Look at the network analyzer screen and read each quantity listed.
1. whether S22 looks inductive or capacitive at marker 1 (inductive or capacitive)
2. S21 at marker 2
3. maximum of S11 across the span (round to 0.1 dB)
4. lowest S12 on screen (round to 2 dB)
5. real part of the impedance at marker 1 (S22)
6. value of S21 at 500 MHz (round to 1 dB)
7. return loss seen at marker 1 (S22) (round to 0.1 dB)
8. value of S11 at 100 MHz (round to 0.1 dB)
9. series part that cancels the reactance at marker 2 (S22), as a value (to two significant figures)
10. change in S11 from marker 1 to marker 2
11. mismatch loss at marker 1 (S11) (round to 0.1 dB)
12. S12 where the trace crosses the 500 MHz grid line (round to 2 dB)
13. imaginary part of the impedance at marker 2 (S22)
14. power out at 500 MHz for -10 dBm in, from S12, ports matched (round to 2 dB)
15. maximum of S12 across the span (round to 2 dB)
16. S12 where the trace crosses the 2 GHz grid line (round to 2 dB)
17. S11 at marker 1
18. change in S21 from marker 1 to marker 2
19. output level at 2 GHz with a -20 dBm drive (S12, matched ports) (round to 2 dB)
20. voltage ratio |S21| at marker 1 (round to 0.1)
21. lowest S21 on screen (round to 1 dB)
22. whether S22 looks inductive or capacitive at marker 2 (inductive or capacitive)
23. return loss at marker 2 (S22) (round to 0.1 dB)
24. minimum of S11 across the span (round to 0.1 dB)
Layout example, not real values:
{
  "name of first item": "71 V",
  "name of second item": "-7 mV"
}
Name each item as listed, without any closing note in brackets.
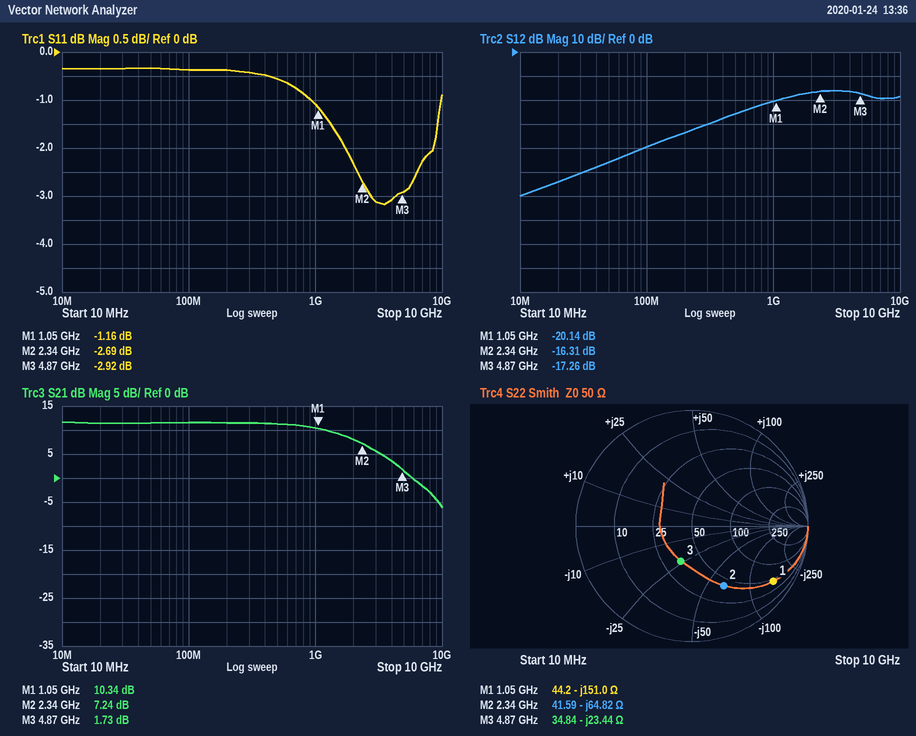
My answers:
{
  "whether S22 looks inductive or capacitive at marker 1": "capacitive",
  "S21 at marker 2": "7.24 dB",
  "maximum of S11 across the span": "-0.3 dB",
  "lowest S12 on screen": "-60 dB",
  "real part of the impedance at marker 1": "44.2 Ω",
  "value of S21 at 500 MHz": "11 dB",
  "return loss seen at marker 1 (S22)": "1.4 dB",
  "value of S11 at 100 MHz": "-0.4 dB",
  "series part that cancels the reactance at marker 2 (S22), as a value": "4.4 nH",
  "change in S11 from marker 1 to marker 2": "-1.53 dB",
  "mismatch loss at marker 1 (S11)": "6.3 dB",
  "S12 where the trace crosses the 500 MHz grid line": "-26 dB",
  "imaginary part of the impedance at marker 2": "-64.82 Ω",
  "power out at 500 MHz for -10 dBm in, from S12, ports matched": "-36 dBm",
  "maximum of S12 across the span": "-16 dB",
  "S12 where the trace crosses the 2 GHz grid line": "-16 dB",
  "S11 at marker 1": "-1.16 dB",
  "change in S21 from marker 1 to marker 2": "-3.10 dB",
  "output level at 2 GHz with a -20 dBm drive (S12, matched ports)": "-36 dBm",
  "voltage ratio |S21| at marker 1": "3.3",
  "lowest S21 on screen": "-6 dB",
  "whether S22 looks inductive or capacitive at marker 2": "capacitive",
  "return loss at marker 2 (S22)": "4.7 dB",
  "minimum of S11 across the span": "-3.2 dB"
}
